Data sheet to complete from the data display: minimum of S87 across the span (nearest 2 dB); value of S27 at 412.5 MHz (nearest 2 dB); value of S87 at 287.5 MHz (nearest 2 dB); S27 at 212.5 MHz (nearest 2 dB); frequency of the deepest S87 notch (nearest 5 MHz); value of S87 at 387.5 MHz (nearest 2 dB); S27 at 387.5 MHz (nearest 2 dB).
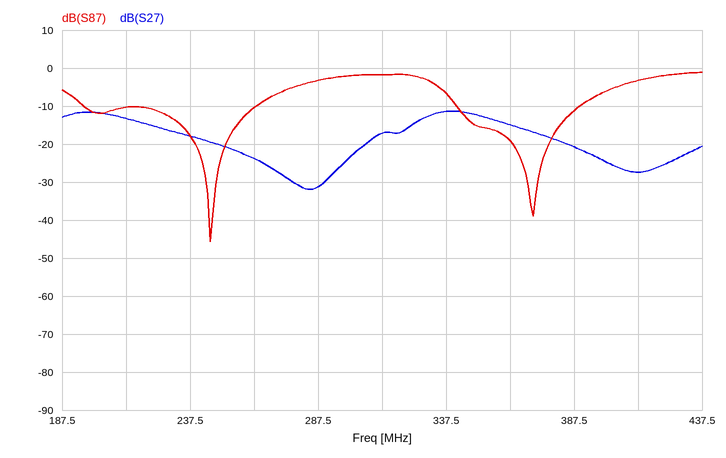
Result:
-46 dB
-28 dB
-4 dB
-14 dB
245 MHz
-12 dB
-20 dB
